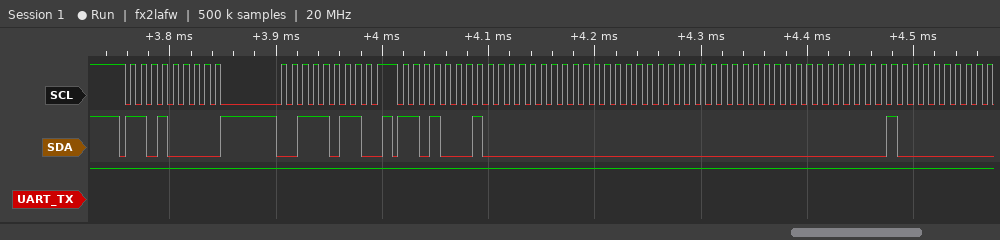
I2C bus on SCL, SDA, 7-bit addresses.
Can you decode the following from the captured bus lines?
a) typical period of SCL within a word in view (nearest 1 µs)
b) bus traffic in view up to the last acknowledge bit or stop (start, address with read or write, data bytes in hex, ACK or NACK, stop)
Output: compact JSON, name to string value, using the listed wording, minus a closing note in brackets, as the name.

{"typical period of SCL within a word in view": "10 µs", "bus traffic in view up to the last acknowledge bit or stop": "start, address 68 write ACK, 3B ACK, stop, start, address 68 read ACK, 00 ACK, 00 ACK, 00 ACK, 00 ACK, 40 ACK"}
